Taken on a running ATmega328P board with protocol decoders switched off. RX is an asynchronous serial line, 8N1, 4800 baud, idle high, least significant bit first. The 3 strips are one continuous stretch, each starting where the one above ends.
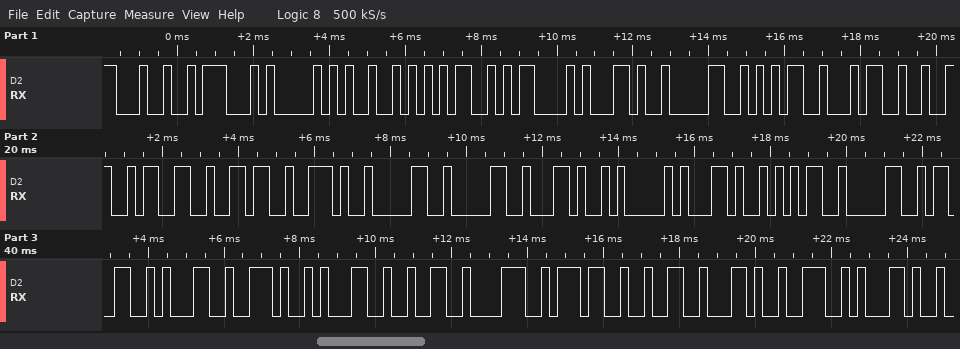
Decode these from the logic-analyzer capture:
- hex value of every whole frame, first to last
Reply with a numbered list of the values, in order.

1. 24 47 50 52 4D 43 2C 30 35 34 32 33 36 2E 30 30 2C 41 2C 35 30 33 31 2E 31 32 38 37 32 2C 4E 2C
